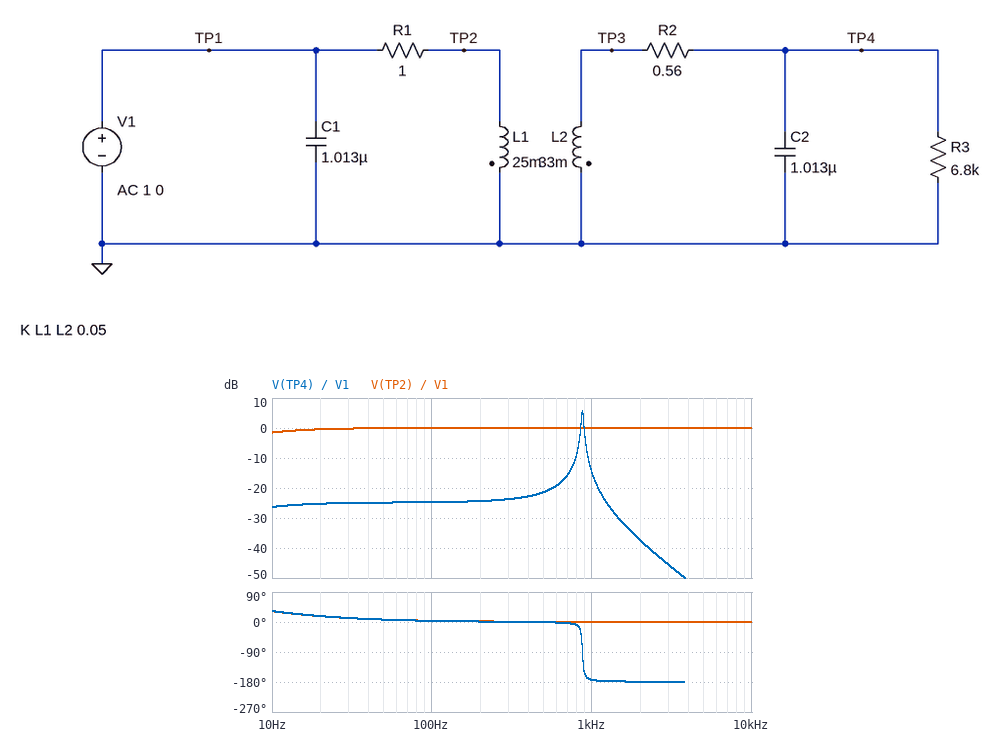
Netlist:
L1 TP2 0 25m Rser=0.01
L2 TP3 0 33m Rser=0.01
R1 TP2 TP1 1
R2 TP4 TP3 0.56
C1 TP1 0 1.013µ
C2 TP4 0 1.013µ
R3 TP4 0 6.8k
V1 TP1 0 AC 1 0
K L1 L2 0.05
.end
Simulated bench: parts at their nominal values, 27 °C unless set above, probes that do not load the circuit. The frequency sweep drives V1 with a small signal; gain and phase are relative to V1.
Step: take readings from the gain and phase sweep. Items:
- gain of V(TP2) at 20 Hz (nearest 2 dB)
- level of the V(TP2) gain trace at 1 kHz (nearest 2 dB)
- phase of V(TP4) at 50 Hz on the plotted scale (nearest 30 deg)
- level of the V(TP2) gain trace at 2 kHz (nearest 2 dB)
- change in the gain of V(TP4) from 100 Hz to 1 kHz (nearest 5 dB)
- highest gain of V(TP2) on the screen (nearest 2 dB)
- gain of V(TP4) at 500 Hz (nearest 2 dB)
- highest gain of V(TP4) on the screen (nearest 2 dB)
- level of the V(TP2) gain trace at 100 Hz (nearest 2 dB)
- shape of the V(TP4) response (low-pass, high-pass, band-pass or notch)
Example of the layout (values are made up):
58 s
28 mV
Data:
0 dB
0 dB
0 deg
0 dB
10 dB
0 dB
-22 dB
6 dB
0 dB
band-pass
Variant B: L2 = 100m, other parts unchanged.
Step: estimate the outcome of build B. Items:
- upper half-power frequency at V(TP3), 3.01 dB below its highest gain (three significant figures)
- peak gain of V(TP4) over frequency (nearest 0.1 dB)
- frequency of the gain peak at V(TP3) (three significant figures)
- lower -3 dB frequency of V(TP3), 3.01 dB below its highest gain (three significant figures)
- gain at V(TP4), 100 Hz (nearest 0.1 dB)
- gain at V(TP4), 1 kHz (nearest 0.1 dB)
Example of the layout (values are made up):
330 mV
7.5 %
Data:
512 Hz
6.4 dB
500 Hz
488 Hz
-19.7 dB
-29.5 dB
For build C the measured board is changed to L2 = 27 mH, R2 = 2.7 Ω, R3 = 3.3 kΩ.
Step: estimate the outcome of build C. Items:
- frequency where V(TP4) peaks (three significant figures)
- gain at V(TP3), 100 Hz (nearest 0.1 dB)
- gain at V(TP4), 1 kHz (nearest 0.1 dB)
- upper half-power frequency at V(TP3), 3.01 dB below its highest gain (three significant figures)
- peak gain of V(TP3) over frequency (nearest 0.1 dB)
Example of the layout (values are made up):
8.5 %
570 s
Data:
963 Hz
-25.6 dB
-5.9 dB
994 Hz
-2.1 dB
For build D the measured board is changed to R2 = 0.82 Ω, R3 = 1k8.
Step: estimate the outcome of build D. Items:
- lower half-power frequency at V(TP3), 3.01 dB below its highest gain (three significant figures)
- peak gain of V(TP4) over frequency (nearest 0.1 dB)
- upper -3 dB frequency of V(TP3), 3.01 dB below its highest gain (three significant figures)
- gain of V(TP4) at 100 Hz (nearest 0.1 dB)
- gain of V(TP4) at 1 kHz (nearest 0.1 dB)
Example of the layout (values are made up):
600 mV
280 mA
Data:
822 Hz
-5.2 dB
914 Hz
-24.7 dB
-15.4 dB
